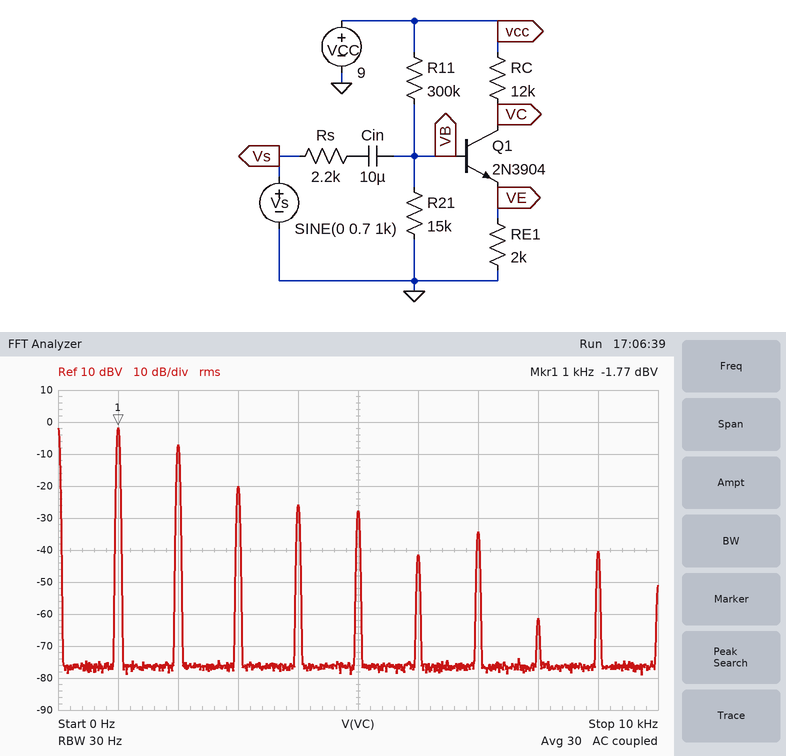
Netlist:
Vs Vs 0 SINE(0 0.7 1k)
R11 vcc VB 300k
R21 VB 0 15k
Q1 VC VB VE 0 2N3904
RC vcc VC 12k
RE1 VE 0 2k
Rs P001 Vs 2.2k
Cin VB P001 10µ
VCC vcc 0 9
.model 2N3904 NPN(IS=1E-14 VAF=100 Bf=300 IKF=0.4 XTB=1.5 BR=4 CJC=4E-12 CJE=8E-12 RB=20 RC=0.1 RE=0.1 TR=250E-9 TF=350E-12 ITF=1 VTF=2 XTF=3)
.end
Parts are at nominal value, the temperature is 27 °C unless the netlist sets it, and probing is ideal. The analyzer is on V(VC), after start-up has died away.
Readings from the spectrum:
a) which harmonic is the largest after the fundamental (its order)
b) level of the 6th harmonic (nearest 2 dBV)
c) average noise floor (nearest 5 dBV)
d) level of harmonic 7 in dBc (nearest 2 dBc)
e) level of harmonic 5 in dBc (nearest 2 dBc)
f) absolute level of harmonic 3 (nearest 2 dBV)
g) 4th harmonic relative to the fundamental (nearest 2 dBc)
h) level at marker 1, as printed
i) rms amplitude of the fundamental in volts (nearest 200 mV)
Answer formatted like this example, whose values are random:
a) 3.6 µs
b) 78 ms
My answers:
a) 2
b) -42 dBV
c) -75 dBV
d) -32 dBc
e) -26 dBc
f) -20 dBV
g) -24 dBc
h) -1.77 dBV
i) 800 mV
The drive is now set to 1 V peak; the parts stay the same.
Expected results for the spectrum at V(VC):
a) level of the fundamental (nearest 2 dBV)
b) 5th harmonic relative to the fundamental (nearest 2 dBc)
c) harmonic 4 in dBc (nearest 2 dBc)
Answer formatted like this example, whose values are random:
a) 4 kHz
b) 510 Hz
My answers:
a) 2 dBV
b) -28 dBc
c) -22 dBc
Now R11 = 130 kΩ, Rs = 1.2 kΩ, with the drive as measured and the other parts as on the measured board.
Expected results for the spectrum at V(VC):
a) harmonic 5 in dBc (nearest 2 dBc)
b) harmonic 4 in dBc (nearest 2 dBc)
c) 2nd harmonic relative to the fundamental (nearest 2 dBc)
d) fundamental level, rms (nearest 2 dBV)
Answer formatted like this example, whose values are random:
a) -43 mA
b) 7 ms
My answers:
a) -44 dBc
b) -36 dBc
c) -16 dBc
d) 6 dBV
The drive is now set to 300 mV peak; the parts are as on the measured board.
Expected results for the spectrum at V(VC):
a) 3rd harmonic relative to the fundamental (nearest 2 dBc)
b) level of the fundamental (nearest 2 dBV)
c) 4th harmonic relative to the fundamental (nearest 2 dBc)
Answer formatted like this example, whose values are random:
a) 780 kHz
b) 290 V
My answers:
a) -12 dBc
b) -14 dBV
c) -38 dBc
